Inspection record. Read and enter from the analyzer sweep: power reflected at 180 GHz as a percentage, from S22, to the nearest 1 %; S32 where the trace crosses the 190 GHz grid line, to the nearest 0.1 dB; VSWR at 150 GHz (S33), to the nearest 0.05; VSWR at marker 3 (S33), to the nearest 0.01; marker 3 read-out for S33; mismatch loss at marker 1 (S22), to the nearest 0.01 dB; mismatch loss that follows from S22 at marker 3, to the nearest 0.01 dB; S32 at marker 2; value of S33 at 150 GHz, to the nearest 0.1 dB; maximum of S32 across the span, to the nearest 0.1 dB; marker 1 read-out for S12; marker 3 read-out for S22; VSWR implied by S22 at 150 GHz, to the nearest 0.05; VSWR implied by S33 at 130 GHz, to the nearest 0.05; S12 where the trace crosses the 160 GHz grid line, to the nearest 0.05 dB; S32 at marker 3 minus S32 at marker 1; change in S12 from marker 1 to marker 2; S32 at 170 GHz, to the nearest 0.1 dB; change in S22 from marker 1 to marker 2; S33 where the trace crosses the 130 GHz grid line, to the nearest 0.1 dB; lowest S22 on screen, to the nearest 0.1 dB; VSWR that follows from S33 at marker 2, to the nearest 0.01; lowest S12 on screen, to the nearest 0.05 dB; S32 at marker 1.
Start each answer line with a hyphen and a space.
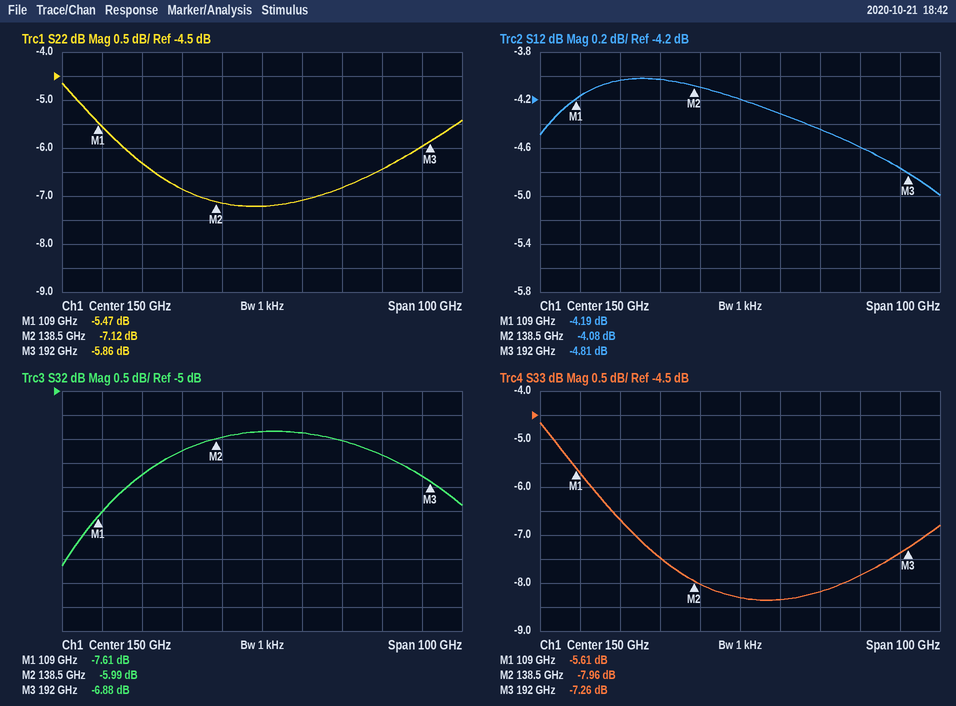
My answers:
- 23 %
- -6.8 dB
- 2.25
- 2.53
- -7.26 dB
- 1.45 dB
- 1.30 dB
- -5.99 dB
- -8.3 dB
- -5.8 dB
- -4.19 dB
- -5.86 dB
- 2.55
- 2.45
- -4.30 dB
- 0.73 dB
- 0.11 dB
- -6.0 dB
- -1.65 dB
- -7.5 dB
- -7.2 dB
- 2.33
- -5.00 dB
- -7.61 dB
